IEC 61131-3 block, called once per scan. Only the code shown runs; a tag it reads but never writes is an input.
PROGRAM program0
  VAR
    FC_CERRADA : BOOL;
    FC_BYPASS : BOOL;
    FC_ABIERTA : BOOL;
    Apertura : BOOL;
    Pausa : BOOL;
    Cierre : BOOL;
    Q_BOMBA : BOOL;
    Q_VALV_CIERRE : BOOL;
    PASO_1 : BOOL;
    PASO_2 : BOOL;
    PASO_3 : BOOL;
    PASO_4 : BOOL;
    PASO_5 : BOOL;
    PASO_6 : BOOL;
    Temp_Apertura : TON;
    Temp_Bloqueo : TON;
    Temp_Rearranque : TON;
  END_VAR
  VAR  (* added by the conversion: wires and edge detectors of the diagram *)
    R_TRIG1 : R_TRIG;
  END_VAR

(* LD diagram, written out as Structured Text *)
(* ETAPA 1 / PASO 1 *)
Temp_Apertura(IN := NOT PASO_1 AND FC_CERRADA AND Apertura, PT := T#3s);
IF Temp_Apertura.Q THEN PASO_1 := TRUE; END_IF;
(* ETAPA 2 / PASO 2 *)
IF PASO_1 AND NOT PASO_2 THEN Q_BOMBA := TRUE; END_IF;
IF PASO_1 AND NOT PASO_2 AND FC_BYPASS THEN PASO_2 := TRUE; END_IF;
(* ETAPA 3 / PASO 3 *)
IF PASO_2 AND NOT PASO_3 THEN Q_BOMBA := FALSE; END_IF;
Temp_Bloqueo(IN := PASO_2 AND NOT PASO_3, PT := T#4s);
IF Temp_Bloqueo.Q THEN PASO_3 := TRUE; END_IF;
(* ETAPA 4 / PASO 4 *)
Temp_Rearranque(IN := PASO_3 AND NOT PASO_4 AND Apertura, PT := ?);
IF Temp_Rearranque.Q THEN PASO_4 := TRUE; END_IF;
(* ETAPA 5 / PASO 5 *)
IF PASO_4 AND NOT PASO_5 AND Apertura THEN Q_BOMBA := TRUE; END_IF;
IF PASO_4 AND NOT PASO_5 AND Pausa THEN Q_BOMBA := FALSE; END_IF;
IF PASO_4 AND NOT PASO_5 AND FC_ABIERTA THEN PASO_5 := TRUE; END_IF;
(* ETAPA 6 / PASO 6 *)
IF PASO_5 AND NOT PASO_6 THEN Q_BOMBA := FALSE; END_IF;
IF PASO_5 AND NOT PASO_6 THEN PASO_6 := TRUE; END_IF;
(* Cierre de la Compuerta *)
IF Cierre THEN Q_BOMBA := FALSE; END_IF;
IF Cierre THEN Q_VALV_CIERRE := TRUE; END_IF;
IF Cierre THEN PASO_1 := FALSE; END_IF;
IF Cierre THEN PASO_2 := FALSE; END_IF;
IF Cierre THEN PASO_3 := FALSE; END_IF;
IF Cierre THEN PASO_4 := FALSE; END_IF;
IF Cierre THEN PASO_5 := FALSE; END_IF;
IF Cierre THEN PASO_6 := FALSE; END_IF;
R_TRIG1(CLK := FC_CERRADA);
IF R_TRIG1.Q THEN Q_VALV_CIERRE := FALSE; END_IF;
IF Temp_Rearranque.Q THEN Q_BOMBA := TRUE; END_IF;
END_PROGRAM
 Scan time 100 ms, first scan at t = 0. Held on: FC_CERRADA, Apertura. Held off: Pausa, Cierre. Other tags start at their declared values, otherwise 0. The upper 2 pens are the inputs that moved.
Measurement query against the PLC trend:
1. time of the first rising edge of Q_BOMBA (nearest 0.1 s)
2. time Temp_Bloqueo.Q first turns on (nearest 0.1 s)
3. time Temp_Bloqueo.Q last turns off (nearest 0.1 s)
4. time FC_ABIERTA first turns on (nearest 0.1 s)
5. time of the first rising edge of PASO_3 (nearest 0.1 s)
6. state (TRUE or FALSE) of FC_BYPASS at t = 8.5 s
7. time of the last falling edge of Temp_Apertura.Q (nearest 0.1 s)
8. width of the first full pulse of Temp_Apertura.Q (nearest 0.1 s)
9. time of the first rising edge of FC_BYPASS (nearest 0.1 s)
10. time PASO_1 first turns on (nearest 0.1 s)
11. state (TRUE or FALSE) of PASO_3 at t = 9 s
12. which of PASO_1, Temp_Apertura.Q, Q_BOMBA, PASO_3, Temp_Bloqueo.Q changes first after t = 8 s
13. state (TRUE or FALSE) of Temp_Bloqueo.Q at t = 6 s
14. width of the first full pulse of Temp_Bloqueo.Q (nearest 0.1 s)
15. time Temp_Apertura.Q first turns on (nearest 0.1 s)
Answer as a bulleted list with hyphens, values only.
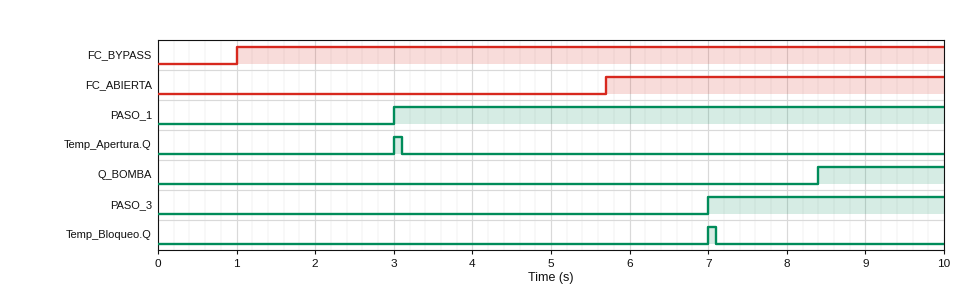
- 8.4 s
- 7.0 s
- 7.1 s
- 5.7 s
- 7.0 s
- TRUE
- 3.1 s
- 0.1 s
- 1.0 s
- 3.0 s
- TRUE
- Q_BOMBA
- FALSE
- 0.1 s
- 3.0 s
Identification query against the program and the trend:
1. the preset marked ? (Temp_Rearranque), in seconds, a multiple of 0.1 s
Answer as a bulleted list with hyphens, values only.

- 1.4 s
